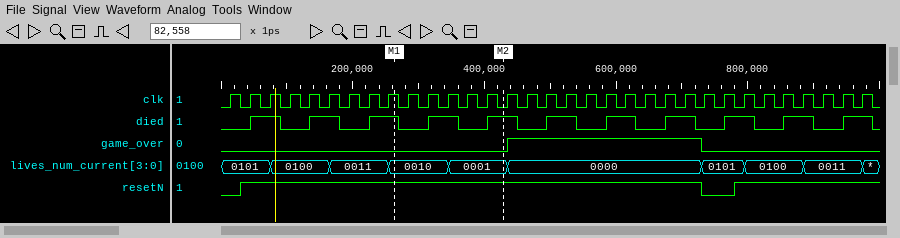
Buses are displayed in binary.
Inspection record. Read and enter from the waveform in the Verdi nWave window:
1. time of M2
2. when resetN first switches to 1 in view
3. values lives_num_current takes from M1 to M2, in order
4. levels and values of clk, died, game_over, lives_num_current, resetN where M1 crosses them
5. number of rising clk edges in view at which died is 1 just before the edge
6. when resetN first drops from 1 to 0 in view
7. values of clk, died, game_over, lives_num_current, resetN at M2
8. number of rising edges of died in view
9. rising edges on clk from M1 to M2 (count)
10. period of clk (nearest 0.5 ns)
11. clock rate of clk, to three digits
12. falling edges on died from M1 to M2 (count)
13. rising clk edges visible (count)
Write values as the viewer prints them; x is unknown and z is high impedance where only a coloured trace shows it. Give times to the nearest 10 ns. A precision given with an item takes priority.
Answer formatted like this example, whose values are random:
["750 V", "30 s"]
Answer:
["430 ns", "30 ns", "0010, 0001", "clk=1, died=1, game_over=0, lives_num_current=0010, resetN=1", "11", "730 ns", "clk=0, died=1, game_over=0, lives_num_current=0001, resetN=1", "11", "5", "30 ns", "33.3 MHz", "2", "33"]
